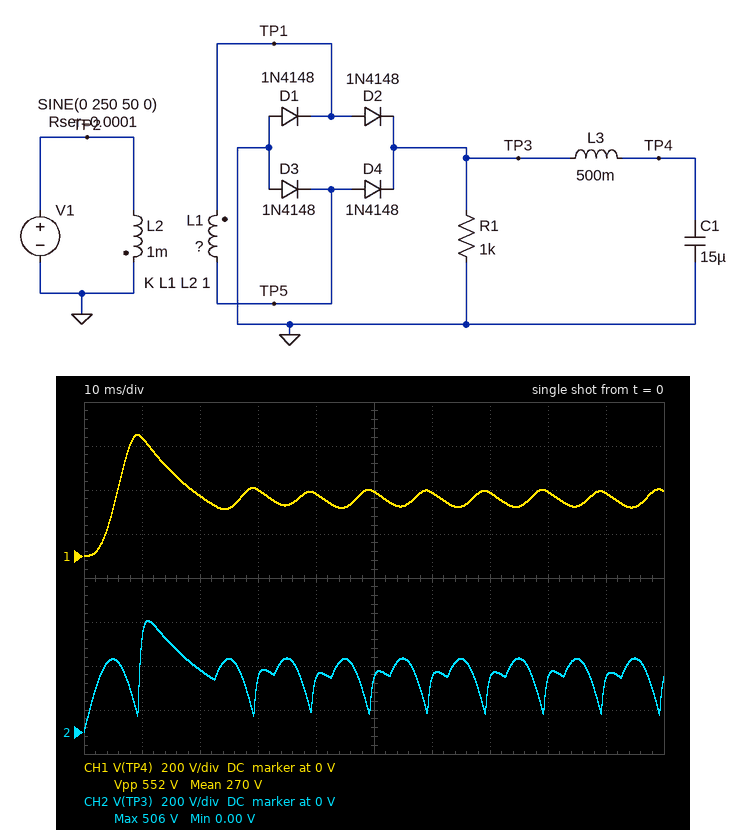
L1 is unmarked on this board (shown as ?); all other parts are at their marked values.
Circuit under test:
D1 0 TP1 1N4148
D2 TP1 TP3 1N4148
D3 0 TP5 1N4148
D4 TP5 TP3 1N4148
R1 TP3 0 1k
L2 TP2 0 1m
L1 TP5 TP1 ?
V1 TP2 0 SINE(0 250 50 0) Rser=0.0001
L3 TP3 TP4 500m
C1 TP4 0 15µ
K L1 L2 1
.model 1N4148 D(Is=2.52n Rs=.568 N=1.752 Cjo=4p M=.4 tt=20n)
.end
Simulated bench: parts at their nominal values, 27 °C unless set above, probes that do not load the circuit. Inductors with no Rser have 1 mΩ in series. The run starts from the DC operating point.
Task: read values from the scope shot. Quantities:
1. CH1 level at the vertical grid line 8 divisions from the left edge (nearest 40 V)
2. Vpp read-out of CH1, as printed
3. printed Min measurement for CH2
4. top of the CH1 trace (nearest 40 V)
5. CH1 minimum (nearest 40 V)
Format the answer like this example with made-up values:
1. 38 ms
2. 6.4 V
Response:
1. 280 V
2. 552 V
3. 0.00 V
4. 560 V
5. 0 V
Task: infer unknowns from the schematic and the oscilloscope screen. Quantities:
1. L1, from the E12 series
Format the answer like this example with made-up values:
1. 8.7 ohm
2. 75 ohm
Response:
1. 1.8 mH
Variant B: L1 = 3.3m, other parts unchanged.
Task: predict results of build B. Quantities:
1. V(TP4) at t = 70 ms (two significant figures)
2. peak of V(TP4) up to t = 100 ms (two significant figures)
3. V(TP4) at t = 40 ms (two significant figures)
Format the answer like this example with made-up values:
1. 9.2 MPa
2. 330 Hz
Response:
1. 390 V
2. 750 V
3. 380 V
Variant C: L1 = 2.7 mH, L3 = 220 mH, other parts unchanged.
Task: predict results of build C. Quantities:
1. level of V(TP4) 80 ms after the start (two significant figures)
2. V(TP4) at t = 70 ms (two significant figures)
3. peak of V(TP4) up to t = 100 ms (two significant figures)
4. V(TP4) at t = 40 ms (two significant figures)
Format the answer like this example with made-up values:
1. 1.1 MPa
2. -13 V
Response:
1. 380 V
2. 390 V
3. 710 V
4. 350 V
